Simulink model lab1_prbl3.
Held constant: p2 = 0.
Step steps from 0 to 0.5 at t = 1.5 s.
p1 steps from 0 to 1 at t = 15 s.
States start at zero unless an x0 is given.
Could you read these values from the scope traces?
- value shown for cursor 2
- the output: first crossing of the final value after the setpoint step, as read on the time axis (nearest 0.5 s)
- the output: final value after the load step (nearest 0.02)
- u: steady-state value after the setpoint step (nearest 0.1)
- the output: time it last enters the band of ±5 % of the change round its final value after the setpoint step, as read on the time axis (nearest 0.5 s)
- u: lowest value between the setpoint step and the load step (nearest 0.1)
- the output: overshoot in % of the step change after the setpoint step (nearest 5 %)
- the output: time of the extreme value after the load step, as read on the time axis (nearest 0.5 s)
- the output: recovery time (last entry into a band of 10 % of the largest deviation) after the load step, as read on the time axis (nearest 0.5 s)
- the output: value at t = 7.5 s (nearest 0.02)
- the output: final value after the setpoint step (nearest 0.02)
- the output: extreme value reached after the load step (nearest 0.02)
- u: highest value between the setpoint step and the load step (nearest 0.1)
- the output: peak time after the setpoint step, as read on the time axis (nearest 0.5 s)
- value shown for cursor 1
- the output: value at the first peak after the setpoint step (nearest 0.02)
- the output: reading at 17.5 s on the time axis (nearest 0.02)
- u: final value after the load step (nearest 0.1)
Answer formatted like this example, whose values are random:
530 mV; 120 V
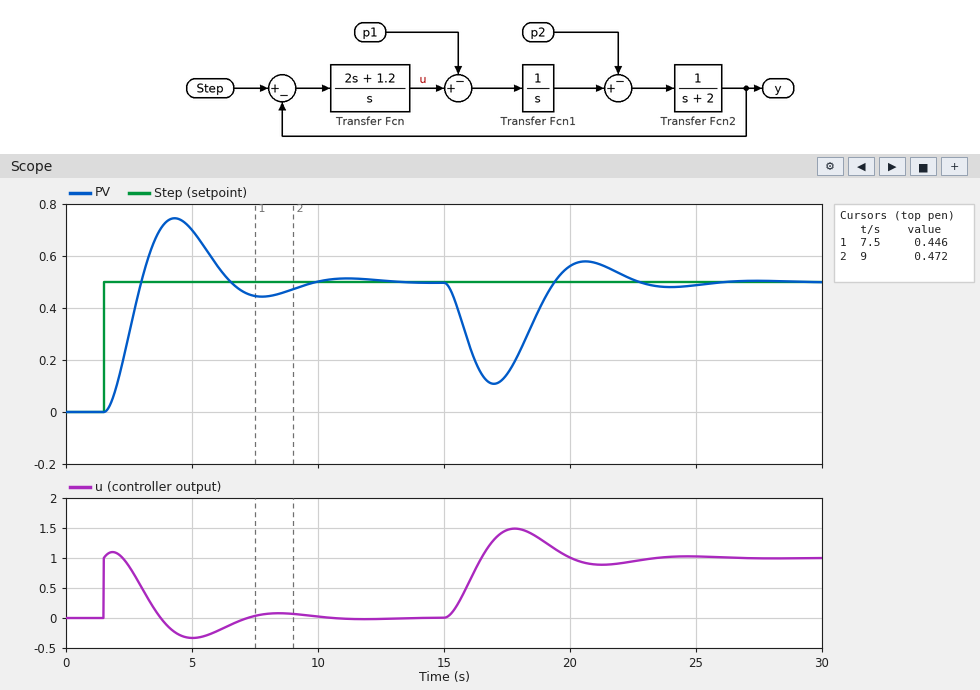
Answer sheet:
0.472; 3.0 s; 0.50; 0.0; 9.0 s; -0.3; 50 %; 17.0 s; 22.0 s; 0.44; 0.50; 0.10; 1.1; 4.5 s; 0.446; 0.74; 0.14; 1.0
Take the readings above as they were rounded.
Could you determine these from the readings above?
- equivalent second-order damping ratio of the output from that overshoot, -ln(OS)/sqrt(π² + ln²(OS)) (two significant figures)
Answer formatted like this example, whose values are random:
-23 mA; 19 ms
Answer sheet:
0.22
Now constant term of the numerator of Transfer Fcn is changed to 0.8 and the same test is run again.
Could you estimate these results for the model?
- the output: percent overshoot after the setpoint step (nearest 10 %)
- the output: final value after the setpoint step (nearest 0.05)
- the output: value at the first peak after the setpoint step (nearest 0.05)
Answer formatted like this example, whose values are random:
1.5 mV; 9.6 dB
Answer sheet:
40 %; 0.50; 0.70
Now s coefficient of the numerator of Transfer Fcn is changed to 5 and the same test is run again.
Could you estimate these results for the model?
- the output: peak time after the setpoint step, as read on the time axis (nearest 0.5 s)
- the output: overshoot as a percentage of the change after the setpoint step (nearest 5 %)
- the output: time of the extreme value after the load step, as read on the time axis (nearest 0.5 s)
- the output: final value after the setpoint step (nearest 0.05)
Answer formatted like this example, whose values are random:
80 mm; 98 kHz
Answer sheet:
3.0 s; 35 %; 16.5 s; 0.50
